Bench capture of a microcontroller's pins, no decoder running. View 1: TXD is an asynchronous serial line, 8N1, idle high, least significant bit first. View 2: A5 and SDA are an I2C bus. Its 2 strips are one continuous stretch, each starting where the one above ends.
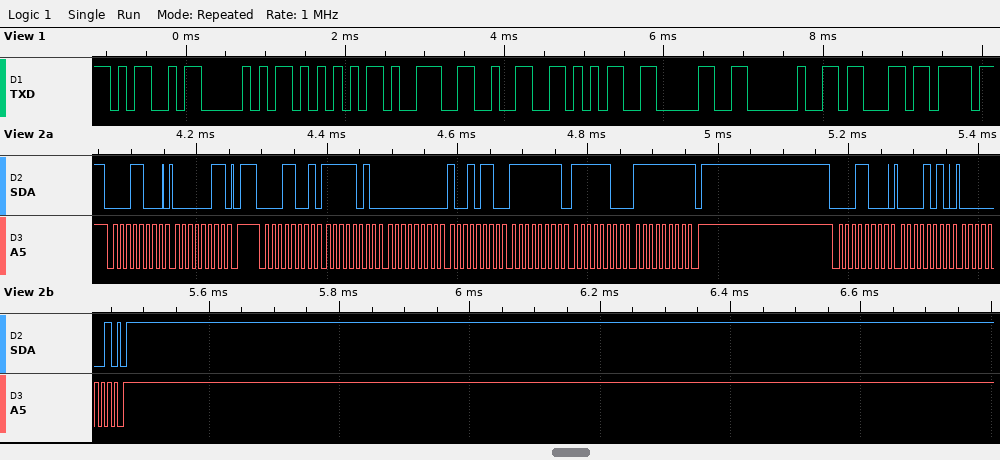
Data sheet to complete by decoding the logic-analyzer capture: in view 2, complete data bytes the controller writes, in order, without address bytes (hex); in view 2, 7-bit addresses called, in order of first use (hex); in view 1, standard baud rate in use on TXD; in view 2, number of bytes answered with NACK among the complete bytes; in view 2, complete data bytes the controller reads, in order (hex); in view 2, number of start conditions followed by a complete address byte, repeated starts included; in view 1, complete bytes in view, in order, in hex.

03 0A 01
0x0C
9600 baud
1
FA 00 96 FF FC FF
3
4D 50 55 39 32 35 30 20 63
